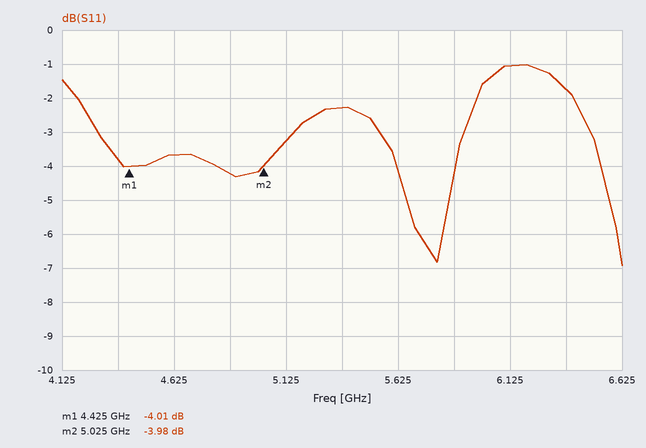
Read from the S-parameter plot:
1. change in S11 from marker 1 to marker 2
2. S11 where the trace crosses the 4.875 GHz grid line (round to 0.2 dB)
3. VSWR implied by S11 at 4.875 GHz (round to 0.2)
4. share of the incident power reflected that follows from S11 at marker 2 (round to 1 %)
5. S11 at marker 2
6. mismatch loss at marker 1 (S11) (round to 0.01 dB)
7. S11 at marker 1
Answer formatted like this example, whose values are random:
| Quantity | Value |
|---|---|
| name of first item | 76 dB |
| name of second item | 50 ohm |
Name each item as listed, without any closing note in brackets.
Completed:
| Quantity | Value |
|---|---|
| change in S11 from marker 1 to marker 2 | 0.03 dB |
| S11 where the trace crosses the 4.875 GHz grid line | -4.2 dB |
| VSWR implied by S11 at 4.875 GHz | 4.2 |
| share of the incident power reflected that follows from S11 at marker 2 | 40 % |
| S11 at marker 2 | -3.98 dB |
| mismatch loss at marker 1 (S11) | 2.20 dB |
| S11 at marker 1 | -4.01 dB |
